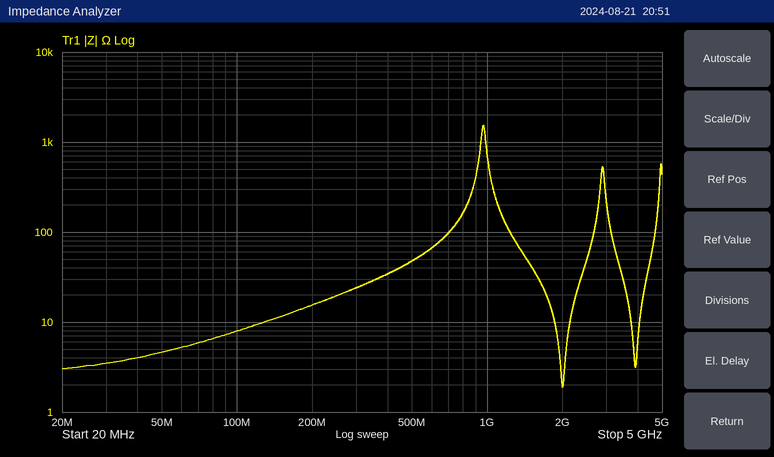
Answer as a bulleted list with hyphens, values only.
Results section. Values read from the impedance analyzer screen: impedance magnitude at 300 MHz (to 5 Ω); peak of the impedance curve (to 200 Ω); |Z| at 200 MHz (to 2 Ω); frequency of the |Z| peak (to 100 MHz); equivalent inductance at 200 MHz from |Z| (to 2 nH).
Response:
- 25 Ω
- 1.6 kΩ
- 16 Ω
- 1.0 GHz
- 12 nH
